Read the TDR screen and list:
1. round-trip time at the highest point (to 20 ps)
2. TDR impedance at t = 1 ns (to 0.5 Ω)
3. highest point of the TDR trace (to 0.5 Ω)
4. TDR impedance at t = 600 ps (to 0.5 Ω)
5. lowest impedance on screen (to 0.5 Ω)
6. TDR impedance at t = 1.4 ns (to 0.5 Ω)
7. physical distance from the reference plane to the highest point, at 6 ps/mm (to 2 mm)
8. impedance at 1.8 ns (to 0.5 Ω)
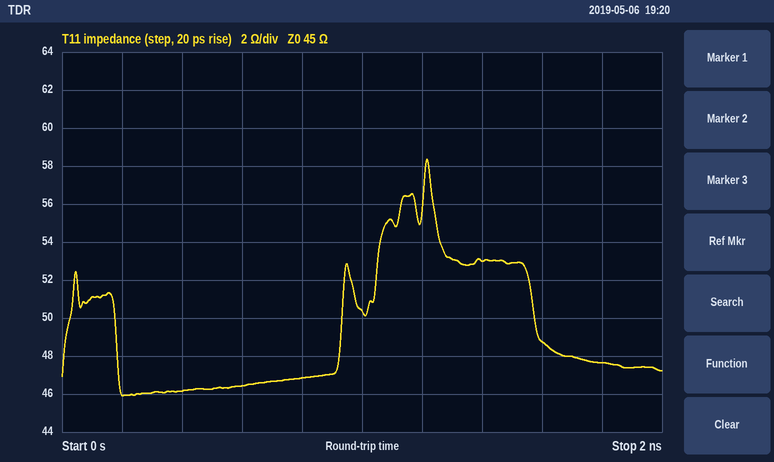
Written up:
1.22 ns
50.5 Ω
58.5 Ω
46.5 Ω
46.0 Ω
53.0 Ω
102 mm
47.5 Ω
